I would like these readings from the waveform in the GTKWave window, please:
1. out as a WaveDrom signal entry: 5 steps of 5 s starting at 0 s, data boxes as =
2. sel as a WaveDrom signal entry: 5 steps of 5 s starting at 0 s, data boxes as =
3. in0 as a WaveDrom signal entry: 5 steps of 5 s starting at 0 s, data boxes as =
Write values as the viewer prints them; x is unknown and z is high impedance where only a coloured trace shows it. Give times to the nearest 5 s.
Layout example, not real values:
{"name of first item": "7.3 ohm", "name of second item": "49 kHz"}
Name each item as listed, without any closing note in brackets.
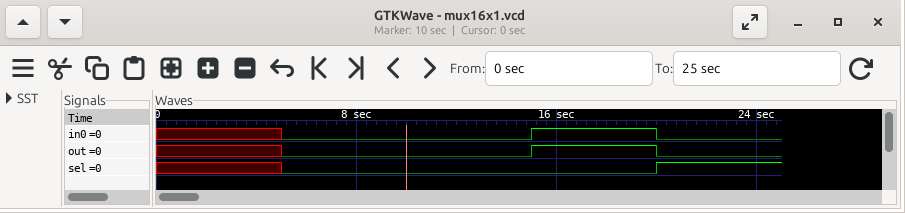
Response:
{"out as a WaveDrom signal entry: 5 steps of 5 s starting at 0 s, data boxes as =": "{name: 'out', wave: 'x0.10'}", "sel as a WaveDrom signal entry: 5 steps of 5 s starting at 0 s, data boxes as =": "{name: 'sel', wave: 'x0..1'}", "in0 as a WaveDrom signal entry: 5 steps of 5 s starting at 0 s, data boxes as =": "{name: 'in0', wave: 'x0.10'}"}
